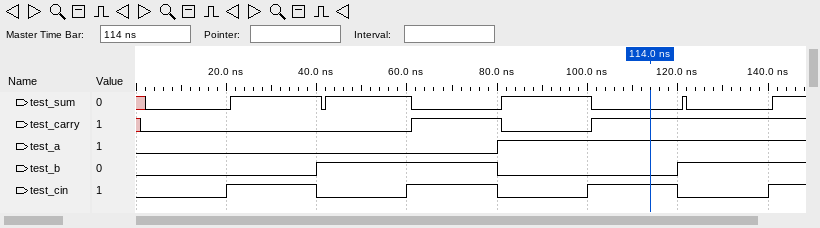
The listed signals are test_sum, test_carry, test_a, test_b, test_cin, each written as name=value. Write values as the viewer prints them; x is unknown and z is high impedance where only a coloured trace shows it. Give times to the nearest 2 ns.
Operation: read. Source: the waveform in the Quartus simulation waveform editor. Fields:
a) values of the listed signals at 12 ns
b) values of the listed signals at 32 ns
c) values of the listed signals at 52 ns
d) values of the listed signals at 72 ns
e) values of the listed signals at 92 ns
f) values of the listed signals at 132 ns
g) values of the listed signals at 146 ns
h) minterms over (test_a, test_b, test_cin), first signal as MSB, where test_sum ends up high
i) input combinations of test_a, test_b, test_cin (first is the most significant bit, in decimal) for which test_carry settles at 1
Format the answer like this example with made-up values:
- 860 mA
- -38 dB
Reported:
- test_sum=0, test_carry=0, test_a=0, test_b=0, test_cin=0
- test_sum=1, test_carry=0, test_a=0, test_b=0, test_cin=1
- test_sum=1, test_carry=0, test_a=0, test_b=1, test_cin=0
- test_sum=0, test_carry=1, test_a=0, test_b=1, test_cin=1
- test_sum=1, test_carry=0, test_a=1, test_b=0, test_cin=0
- test_sum=0, test_carry=1, test_a=1, test_b=1, test_cin=0
- test_sum=1, test_carry=1, test_a=1, test_b=1, test_cin=1
- 1, 2, 4, 7
- 3, 5, 6, 7
